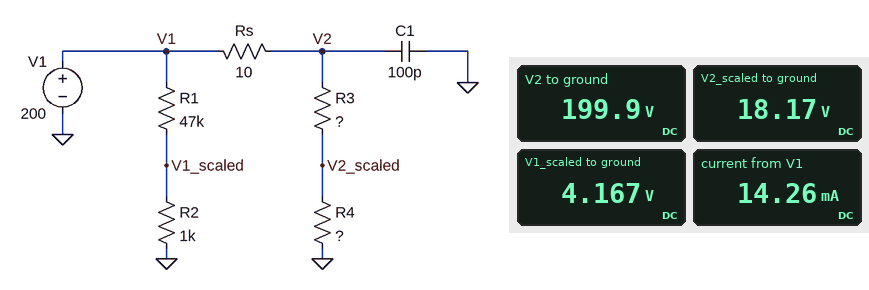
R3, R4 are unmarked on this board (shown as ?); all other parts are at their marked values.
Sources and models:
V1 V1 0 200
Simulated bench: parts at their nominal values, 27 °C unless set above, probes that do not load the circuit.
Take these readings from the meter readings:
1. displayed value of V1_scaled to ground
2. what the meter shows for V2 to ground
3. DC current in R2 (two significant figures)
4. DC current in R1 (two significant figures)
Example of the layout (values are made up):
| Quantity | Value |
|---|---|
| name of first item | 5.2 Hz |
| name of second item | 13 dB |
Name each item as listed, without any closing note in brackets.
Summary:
| Quantity | Value |
|---|---|
| displayed value of V1_scaled to ground | 4.167 V |
| what the meter shows for V2 to ground | 199.9 V |
| DC current in R2 | 4.2 mA |
| DC current in R1 | 4.2 mA |
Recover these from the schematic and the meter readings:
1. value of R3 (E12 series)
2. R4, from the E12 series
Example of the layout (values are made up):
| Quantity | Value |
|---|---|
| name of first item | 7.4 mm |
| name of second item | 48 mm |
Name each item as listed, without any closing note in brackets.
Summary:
| Quantity | Value |
|---|---|
| value of R3 | 18 kΩ |
| R4, from the E12 series | 1.8 kΩ |
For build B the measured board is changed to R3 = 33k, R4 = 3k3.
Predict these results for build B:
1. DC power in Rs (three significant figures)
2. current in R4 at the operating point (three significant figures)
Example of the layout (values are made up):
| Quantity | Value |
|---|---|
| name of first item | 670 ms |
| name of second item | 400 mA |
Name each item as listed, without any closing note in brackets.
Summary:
| Quantity | Value |
|---|---|
| DC power in Rs | 303 µW |
| current in R4 at the operating point | 5.51 mA |
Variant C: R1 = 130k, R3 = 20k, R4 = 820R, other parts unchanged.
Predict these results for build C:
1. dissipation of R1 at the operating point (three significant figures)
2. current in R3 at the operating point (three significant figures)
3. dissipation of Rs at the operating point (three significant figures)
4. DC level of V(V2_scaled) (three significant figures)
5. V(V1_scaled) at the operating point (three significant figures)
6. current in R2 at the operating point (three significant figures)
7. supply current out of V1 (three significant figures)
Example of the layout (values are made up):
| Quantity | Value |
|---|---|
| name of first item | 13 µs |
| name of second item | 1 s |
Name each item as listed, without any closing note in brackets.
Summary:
| Quantity | Value |
|---|---|
| dissipation of R1 at the operating point | 303 mW |
| current in R3 at the operating point | 9.60 mA |
| dissipation of Rs at the operating point | 922 µW |
| DC level of V(V2_scaled) | 7.87 V |
| V(V1_scaled) at the operating point | 1.53 V |
| current in R2 at the operating point | 1.53 mA |
| supply current out of V1 | 11.1 mA |
